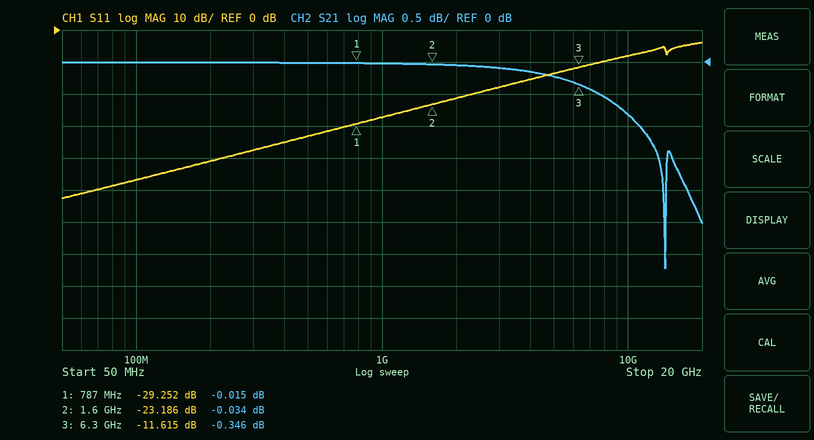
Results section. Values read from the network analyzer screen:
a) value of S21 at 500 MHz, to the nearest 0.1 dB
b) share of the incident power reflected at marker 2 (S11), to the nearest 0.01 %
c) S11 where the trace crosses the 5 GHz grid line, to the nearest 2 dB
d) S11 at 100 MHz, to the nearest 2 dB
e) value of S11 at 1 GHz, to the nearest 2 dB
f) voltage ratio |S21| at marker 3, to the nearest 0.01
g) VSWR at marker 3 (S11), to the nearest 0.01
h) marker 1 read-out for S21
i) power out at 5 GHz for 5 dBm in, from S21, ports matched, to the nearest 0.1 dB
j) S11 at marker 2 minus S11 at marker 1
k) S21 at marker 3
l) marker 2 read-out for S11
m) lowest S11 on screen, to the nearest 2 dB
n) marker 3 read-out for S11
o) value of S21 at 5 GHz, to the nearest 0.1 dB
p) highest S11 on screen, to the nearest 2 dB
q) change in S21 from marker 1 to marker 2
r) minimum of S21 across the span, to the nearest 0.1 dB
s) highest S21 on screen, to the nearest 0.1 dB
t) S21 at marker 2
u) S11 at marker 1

0.0 dB
0.48 %
-14 dB
-46 dB
-28 dB
0.96
1.71
-0.015 dB
4.8 dBm
6.066 dB
-0.346 dB
-23.186 dB
-52 dB
-11.615 dB
-0.2 dB
-4 dB
-0.019 dB
-3.2 dB
0.0 dB
-0.034 dB
-29.252 dB
